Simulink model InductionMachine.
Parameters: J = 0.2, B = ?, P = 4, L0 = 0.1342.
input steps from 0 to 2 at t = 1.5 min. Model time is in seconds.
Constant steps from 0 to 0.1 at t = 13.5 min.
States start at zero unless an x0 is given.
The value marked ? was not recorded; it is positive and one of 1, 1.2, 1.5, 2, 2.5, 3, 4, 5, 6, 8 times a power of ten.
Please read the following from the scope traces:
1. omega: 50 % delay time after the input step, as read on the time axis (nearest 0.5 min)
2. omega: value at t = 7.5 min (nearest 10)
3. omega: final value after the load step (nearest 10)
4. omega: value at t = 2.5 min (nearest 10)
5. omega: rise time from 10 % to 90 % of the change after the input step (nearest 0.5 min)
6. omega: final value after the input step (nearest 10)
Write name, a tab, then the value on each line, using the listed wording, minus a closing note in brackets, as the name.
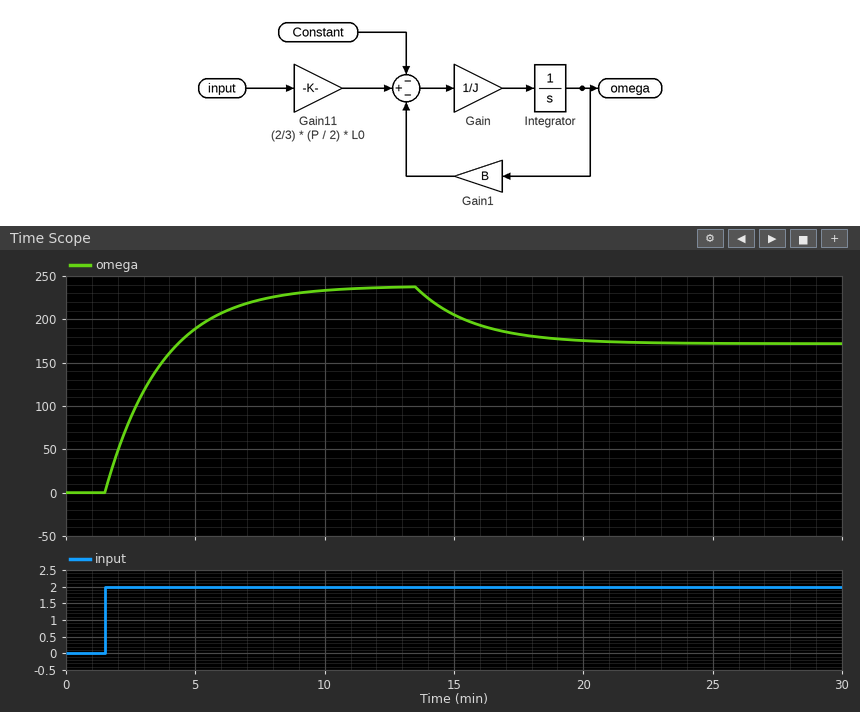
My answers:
omega: 50 % delay time after the input step, as read on the time axis	3.0 min
omega: value at t = 7.5 min	220
omega: final value after the load step	170
omega: value at t = 2.5 min	90
omega: rise time from 10 % to 90 % of the change after the input step	5.0 min
omega: final value after the input step	240
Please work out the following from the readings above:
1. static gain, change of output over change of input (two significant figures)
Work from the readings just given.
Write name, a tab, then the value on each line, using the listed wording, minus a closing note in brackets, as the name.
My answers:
static gain, change of output over change of input	120
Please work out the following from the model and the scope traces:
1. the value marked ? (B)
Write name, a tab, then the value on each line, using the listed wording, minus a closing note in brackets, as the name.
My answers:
the value marked ?	0.0015
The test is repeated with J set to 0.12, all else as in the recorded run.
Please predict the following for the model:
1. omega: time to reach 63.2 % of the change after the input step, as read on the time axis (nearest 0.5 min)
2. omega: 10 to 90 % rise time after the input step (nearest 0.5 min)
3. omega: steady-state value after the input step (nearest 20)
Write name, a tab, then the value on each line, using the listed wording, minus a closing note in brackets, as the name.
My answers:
omega: time to reach 63.2 % of the change after the input step, as read on the time axis	3.0 min
omega: 10 to 90 % rise time after the input step	3.0 min
omega: steady-state value after the input step	240
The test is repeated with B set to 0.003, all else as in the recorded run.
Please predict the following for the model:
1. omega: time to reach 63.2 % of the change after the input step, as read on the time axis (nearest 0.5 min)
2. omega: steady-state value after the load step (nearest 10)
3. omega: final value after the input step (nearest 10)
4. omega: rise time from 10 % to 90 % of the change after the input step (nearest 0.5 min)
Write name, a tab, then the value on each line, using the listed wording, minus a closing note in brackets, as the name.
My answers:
omega: time to reach 63.2 % of the change after the input step, as read on the time axis	2.5 min
omega: steady-state value after the load step	90
omega: final value after the input step	120
omega: rise time from 10 % to 90 % of the change after the input step	2.5 min
